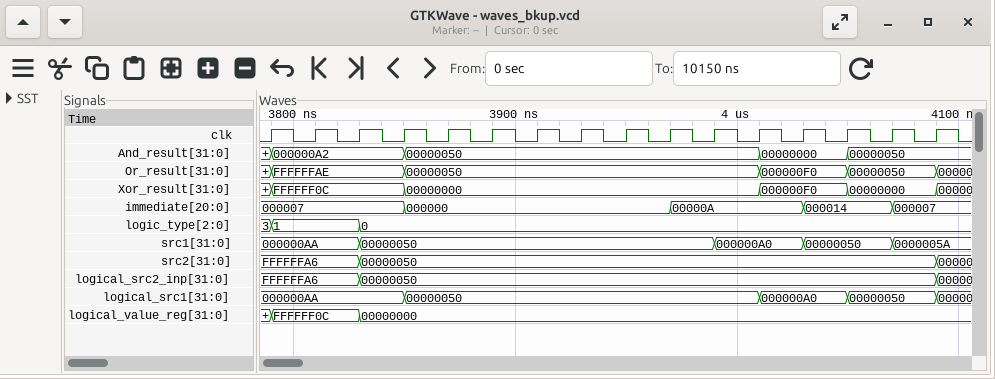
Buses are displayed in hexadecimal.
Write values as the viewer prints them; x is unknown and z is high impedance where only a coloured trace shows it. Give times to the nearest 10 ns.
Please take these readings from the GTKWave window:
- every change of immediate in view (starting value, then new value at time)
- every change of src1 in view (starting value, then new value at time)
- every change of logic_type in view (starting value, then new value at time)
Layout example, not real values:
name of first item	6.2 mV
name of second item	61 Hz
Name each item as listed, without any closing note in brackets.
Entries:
every change of immediate in view	000007, 000000 at 3850 ns, 00000A at 3970 ns, 000014 at 4030 ns, 000007 at 4070 ns
every change of src1 in view	000000AA, 00000050 at 3830 ns, 000000A0 at 3990 ns, 00000050 at 4030 ns, 0000005A at 4070 ns
every change of logic_type in view	3, 1 at 3790 ns, 0 at 3830 ns
